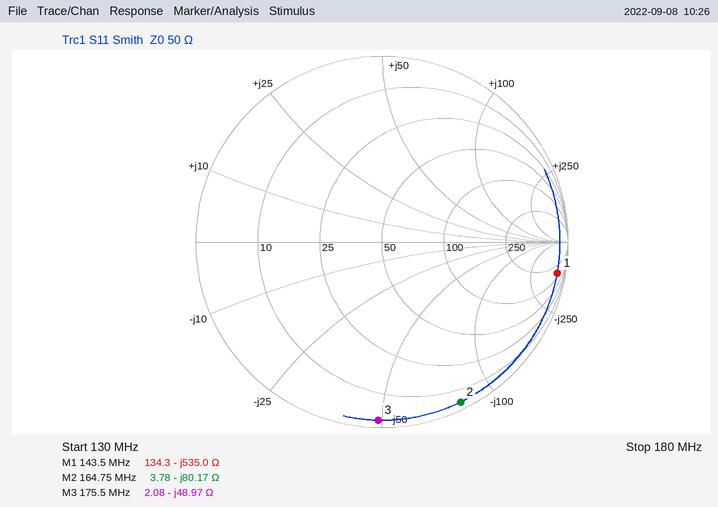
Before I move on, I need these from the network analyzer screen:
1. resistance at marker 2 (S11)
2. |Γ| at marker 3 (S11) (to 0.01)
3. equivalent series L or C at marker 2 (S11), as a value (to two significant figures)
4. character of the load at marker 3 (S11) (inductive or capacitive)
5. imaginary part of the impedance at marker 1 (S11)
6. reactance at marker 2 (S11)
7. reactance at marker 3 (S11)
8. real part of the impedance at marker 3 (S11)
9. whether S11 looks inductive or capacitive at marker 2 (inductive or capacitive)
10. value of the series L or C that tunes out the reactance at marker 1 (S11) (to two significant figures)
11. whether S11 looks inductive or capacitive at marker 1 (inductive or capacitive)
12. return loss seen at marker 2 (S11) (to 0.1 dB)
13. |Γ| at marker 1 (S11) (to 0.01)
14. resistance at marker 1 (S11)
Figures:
3.78 Ω
0.96
12 pF
capacitive
-535.0 Ω
-80.17 Ω
-48.97 Ω
2.08 Ω
capacitive
590 nH
capacitive
0.4 dB
0.96
134.3 Ω
